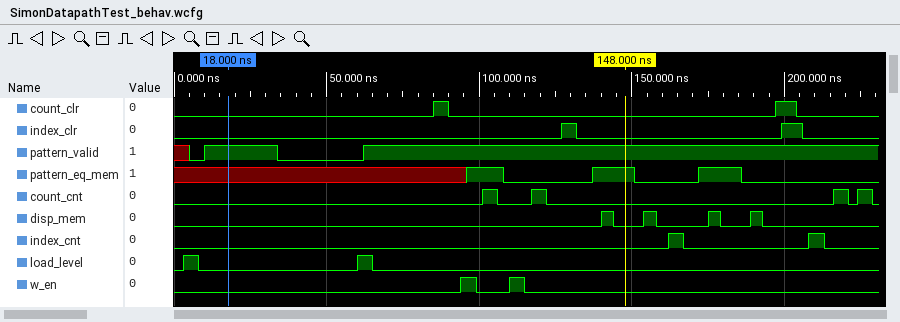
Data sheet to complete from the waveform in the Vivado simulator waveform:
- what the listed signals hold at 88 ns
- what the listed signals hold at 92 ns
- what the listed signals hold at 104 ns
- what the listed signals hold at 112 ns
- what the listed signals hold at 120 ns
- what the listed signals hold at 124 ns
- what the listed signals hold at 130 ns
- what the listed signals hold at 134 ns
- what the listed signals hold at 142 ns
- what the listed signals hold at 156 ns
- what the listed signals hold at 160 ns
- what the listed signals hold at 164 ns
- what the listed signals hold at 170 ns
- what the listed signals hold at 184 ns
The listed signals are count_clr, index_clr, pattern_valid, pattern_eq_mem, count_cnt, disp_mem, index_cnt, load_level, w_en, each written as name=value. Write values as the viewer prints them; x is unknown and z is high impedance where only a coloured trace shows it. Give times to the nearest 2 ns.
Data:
count_clr=1, index_clr=0, pattern_valid=1, pattern_eq_mem=x, count_cnt=0, disp_mem=0, index_cnt=0, load_level=0, w_en=0
count_clr=0, index_clr=0, pattern_valid=1, pattern_eq_mem=x, count_cnt=0, disp_mem=0, index_cnt=0, load_level=0, w_en=0
count_clr=0, index_clr=0, pattern_valid=1, pattern_eq_mem=1, count_cnt=1, disp_mem=0, index_cnt=0, load_level=0, w_en=0
count_clr=0, index_clr=0, pattern_valid=1, pattern_eq_mem=0, count_cnt=0, disp_mem=0, index_cnt=0, load_level=0, w_en=1
count_clr=0, index_clr=0, pattern_valid=1, pattern_eq_mem=0, count_cnt=1, disp_mem=0, index_cnt=0, load_level=0, w_en=0
count_clr=0, index_clr=0, pattern_valid=1, pattern_eq_mem=0, count_cnt=0, disp_mem=0, index_cnt=0, load_level=0, w_en=0
count_clr=0, index_clr=1, pattern_valid=1, pattern_eq_mem=0, count_cnt=0, disp_mem=0, index_cnt=0, load_level=0, w_en=0
count_clr=0, index_clr=0, pattern_valid=1, pattern_eq_mem=0, count_cnt=0, disp_mem=0, index_cnt=0, load_level=0, w_en=0
count_clr=0, index_clr=0, pattern_valid=1, pattern_eq_mem=1, count_cnt=0, disp_mem=1, index_cnt=0, load_level=0, w_en=0
count_clr=0, index_clr=0, pattern_valid=1, pattern_eq_mem=0, count_cnt=0, disp_mem=1, index_cnt=0, load_level=0, w_en=0
count_clr=0, index_clr=0, pattern_valid=1, pattern_eq_mem=0, count_cnt=0, disp_mem=0, index_cnt=0, load_level=0, w_en=0
count_clr=0, index_clr=0, pattern_valid=1, pattern_eq_mem=0, count_cnt=0, disp_mem=0, index_cnt=1, load_level=0, w_en=0
count_clr=0, index_clr=0, pattern_valid=1, pattern_eq_mem=0, count_cnt=0, disp_mem=0, index_cnt=0, load_level=0, w_en=0
count_clr=0, index_clr=0, pattern_valid=1, pattern_eq_mem=1, count_cnt=0, disp_mem=0, index_cnt=0, load_level=0, w_en=0
